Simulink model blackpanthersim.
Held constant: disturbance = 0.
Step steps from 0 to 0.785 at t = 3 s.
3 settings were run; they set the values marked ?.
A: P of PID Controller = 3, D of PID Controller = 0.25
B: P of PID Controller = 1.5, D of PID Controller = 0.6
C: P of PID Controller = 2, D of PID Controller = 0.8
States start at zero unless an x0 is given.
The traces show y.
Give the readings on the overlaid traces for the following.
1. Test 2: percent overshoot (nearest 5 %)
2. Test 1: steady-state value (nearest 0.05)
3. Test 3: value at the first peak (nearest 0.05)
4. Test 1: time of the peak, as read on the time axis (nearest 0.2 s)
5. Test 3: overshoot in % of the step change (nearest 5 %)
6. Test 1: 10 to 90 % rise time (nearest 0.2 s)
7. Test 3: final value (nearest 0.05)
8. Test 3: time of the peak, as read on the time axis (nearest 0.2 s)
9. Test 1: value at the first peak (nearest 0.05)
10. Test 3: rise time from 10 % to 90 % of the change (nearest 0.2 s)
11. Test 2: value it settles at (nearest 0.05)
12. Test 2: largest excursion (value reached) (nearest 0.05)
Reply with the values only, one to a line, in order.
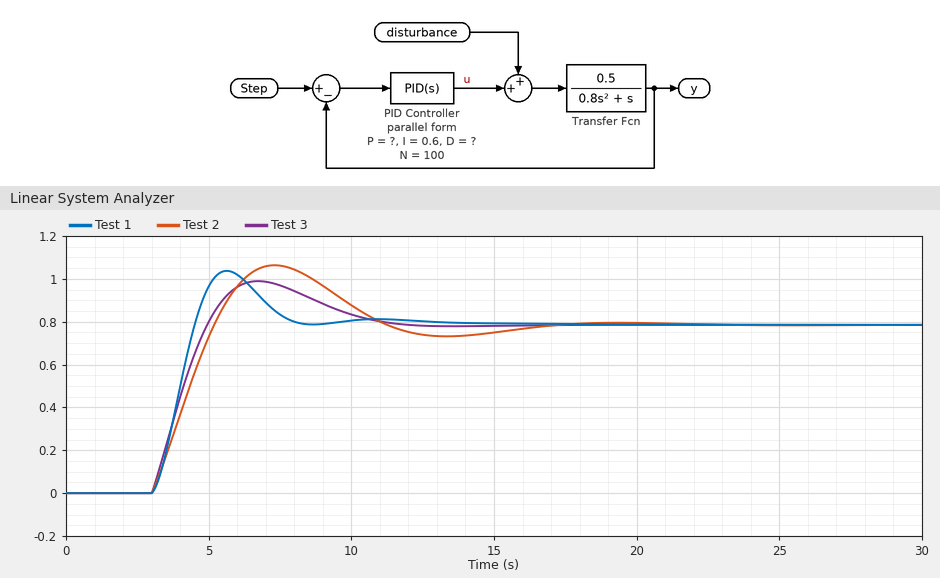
35 %
0.80
1.00
5.6 s
25 %
1.0 s
0.80
6.8 s
1.05
1.4 s
0.80
1.05
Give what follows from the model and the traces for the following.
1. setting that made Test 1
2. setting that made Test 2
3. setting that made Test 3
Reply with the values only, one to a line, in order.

A
B
C
